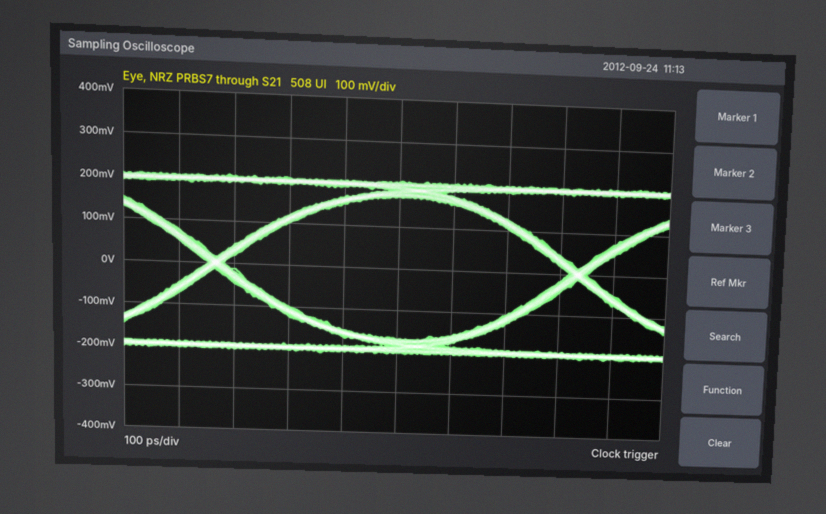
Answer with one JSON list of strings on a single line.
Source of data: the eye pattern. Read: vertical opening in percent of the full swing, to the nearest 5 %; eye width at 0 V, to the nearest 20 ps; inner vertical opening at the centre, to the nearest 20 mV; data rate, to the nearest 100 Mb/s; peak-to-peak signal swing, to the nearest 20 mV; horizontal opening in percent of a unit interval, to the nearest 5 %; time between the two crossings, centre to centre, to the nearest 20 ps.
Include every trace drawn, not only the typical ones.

["80 %", "640 ps", "340 mV", "1.5 Gb/s", "420 mV", "95 %", "660 ps"]
